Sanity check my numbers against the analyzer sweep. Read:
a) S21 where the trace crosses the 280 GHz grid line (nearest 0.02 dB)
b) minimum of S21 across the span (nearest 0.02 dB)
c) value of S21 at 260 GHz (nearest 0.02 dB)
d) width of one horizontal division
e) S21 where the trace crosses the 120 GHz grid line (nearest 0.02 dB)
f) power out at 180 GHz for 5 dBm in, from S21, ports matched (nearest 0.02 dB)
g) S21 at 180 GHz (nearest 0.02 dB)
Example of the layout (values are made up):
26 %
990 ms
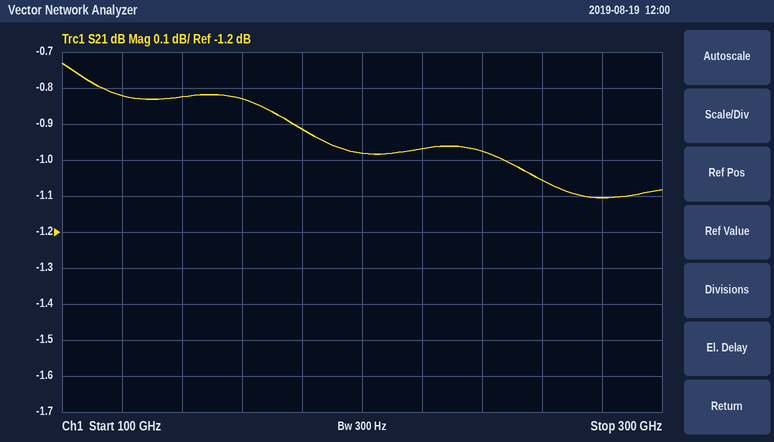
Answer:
-1.10 dB
-1.10 dB
-1.06 dB
20 GHz
-0.82 dB
4.08 dBm
-0.92 dB
